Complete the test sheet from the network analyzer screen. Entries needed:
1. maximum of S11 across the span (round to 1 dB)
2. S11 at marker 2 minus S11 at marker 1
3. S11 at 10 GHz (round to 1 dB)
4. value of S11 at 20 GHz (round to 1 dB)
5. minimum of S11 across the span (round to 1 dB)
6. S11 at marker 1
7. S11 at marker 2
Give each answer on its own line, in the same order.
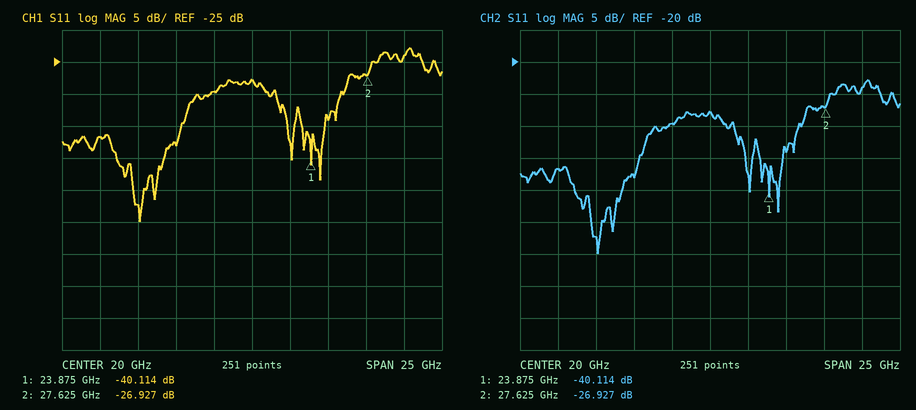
-23 dB
13.187 dB
-37 dB
-28 dB
-50 dB
-40.114 dB
-26.927 dB
